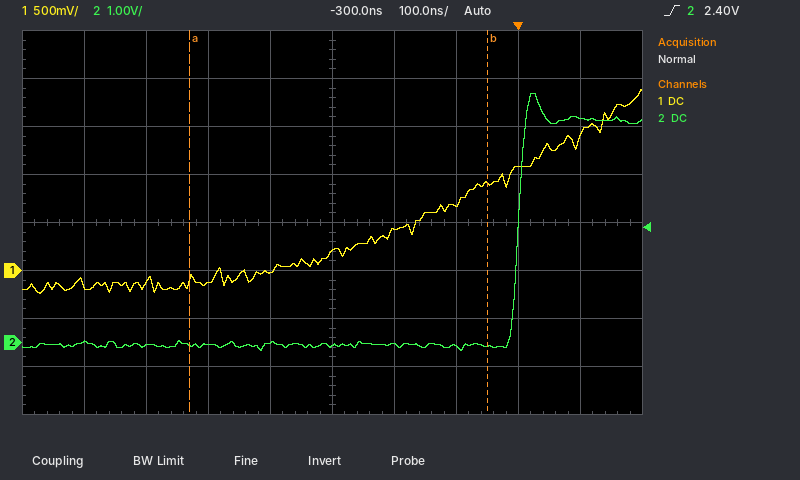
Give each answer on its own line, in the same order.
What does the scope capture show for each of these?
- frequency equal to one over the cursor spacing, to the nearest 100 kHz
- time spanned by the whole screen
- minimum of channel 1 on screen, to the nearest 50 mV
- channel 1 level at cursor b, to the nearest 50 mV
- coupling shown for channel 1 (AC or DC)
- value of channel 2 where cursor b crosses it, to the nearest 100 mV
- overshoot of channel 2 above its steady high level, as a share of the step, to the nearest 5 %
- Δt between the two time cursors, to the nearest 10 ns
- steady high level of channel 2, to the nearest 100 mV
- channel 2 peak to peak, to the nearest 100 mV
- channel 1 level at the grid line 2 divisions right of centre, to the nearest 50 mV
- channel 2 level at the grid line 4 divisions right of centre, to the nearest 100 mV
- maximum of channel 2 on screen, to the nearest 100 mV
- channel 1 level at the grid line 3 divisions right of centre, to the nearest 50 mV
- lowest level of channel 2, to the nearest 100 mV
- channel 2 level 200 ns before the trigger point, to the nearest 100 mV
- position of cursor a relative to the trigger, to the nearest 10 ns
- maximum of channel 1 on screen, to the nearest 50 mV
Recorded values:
2.1 MHz
1 µs
-250 mV
900 mV
DC
-100 mV
10 %
480 ns
4.6 V
5.4 V
700 mV
4.7 V
5.2 V
1.10 V
-200 mV
0.0 V
-530 ns
1.90 V
